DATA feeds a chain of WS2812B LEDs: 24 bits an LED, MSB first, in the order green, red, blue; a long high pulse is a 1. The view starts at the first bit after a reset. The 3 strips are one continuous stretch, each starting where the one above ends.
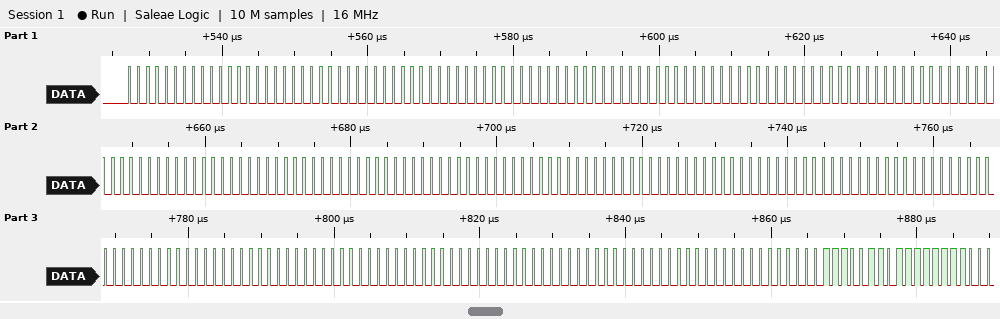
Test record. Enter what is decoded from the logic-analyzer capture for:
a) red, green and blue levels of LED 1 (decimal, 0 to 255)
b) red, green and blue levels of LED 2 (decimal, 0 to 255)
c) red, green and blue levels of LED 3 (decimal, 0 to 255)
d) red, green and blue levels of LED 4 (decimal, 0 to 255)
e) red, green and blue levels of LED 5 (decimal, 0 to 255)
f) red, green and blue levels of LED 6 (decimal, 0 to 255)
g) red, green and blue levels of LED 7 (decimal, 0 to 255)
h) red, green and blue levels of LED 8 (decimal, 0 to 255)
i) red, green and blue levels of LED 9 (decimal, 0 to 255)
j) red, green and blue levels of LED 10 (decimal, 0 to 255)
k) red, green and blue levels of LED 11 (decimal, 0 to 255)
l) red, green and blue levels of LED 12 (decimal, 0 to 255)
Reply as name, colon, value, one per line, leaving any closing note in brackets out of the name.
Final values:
red, green and blue levels of LED 1: 0, 0, 0
red, green and blue levels of LED 2: 0, 0, 0
red, green and blue levels of LED 3: 0, 0, 0
red, green and blue levels of LED 4: 0, 0, 0
red, green and blue levels of LED 5: 0, 0, 0
red, green and blue levels of LED 6: 0, 0, 0
red, green and blue levels of LED 7: 0, 0, 0
red, green and blue levels of LED 8: 0, 0, 0
red, green and blue levels of LED 9: 0, 0, 0
red, green and blue levels of LED 10: 0, 0, 0
red, green and blue levels of LED 11: 0, 0, 0
red, green and blue levels of LED 12: 230, 0, 255
